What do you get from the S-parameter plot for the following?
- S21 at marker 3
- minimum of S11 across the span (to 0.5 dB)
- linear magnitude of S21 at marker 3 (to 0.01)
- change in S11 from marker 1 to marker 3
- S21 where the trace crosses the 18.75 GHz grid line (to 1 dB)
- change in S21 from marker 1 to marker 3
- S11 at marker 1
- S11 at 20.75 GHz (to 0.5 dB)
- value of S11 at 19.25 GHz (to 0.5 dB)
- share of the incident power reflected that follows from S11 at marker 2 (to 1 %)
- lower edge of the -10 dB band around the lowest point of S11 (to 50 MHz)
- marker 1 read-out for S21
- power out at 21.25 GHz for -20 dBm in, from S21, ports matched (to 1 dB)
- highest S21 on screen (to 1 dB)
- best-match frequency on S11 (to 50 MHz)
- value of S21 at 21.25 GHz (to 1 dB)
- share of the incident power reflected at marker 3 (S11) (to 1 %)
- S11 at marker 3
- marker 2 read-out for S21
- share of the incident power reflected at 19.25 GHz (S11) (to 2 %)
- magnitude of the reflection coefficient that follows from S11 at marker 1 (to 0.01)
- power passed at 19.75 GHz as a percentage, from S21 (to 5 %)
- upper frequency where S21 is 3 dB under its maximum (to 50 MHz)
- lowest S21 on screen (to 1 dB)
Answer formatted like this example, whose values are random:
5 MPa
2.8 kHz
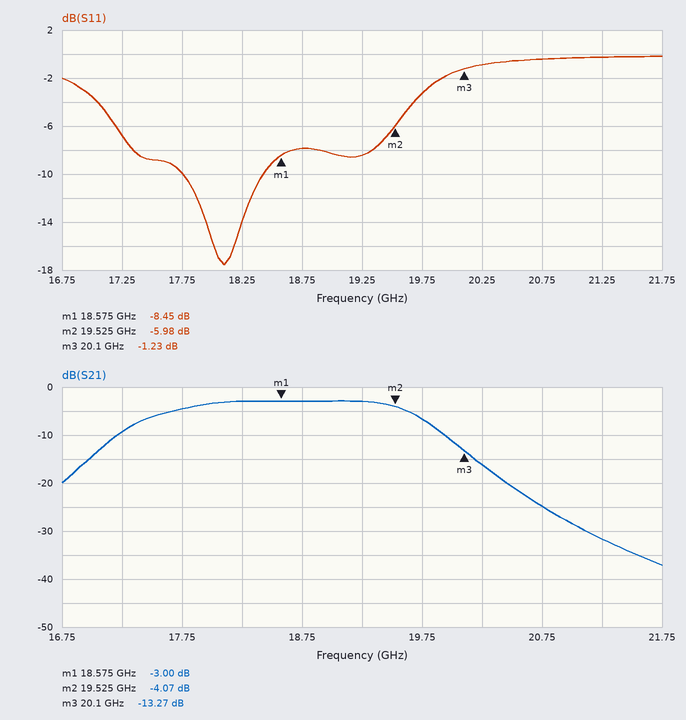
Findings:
-13.27 dB
-17.5 dB
0.22
7.22 dB
-3 dB
-10.27 dB
-8.45 dB
-0.5 dB
-8.5 dB
25 %
17.75 GHz
-3.00 dB
-52 dBm
-3 dB
18.10 GHz
-32 dB
75 %
-1.23 dB
-4.07 dB
14 %
0.38
20 %
19.70 GHz
-37 dB
